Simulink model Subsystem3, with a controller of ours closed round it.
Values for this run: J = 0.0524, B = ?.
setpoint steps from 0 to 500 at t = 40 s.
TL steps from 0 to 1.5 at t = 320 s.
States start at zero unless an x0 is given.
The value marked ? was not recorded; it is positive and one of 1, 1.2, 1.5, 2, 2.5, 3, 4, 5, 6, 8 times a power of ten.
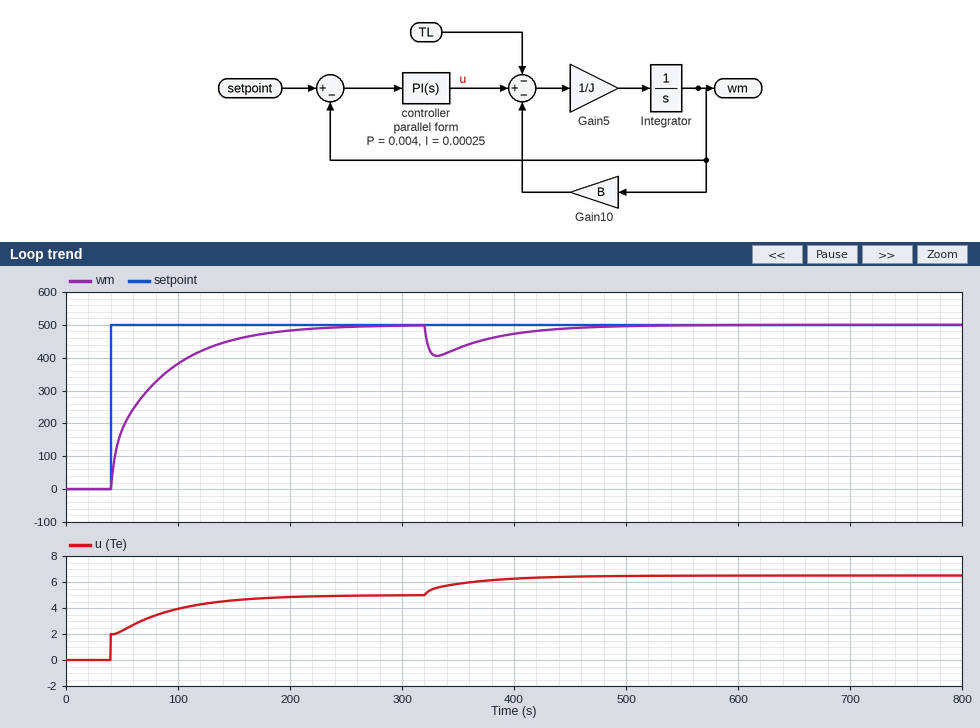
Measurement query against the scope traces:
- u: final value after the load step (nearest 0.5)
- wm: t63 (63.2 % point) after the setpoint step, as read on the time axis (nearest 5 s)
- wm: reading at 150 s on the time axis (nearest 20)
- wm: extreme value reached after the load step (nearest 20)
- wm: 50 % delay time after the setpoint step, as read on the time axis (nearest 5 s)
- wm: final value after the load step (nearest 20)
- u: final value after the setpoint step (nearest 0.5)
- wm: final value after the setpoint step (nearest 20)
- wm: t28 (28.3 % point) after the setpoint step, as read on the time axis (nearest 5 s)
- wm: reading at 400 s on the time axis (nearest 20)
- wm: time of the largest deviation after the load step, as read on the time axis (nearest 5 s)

6.5
75 s
460
400
60 s
500
5.0
500
45 s
480
330 s
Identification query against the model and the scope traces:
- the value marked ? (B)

0.01
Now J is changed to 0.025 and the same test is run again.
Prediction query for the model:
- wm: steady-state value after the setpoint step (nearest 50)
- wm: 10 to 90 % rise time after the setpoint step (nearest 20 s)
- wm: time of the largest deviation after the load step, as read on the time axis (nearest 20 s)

500
100 s
320 s
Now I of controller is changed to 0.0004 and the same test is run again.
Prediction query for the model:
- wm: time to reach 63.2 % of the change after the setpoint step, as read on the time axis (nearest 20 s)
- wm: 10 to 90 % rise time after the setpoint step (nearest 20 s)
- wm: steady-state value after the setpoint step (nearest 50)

60 s
60 s
500
